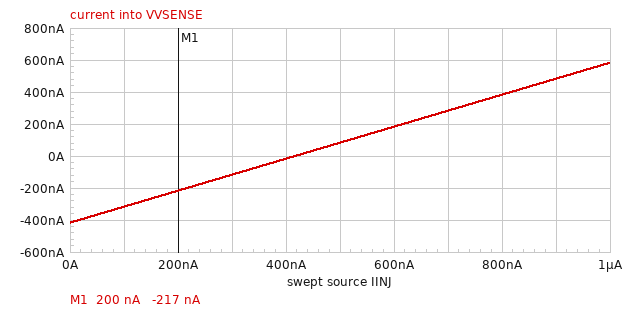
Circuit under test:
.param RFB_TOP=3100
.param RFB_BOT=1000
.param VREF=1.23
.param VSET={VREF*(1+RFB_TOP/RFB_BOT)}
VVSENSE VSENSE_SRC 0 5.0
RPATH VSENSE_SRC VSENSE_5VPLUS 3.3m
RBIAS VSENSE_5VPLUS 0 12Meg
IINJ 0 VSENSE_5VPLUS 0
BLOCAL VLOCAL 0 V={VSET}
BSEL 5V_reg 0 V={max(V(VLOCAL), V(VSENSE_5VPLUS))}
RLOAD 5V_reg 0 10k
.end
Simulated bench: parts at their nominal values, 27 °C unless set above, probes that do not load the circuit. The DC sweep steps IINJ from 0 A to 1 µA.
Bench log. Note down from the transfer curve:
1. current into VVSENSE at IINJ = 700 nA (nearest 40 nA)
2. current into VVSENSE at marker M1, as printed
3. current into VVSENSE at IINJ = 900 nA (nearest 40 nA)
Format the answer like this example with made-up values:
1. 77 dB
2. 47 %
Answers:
1. 280 nA
2. -217 nA
3. 480 nA
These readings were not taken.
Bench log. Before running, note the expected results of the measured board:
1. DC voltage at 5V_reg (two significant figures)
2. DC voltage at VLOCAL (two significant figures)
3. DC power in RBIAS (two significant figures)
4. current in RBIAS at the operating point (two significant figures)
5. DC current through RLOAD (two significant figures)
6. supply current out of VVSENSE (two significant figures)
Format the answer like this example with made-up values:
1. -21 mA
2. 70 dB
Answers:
1. 5.0 V
2. 5.0 V
3. 2.1 µW
4. 420 nA
5. 500 µA
6. 420 nA
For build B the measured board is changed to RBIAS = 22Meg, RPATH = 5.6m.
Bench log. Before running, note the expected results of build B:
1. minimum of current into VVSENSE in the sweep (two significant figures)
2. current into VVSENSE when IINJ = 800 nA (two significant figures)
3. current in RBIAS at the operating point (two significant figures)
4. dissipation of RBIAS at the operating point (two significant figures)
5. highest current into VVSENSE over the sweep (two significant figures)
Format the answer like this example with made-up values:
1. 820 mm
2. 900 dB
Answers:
1. -230 nA
2. 570 nA
3. 230 nA
4. 1.1 µW
5. 770 nA
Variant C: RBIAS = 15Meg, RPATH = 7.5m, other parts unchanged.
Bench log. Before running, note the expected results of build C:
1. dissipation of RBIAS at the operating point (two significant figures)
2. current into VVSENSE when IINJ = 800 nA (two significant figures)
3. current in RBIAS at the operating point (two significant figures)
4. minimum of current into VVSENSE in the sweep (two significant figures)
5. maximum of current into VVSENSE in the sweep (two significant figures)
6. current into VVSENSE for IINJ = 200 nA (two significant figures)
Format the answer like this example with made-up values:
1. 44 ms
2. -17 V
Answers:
1. 1.7 µW
2. 470 nA
3. 330 nA
4. -330 nA
5. 670 nA
6. -130 nA
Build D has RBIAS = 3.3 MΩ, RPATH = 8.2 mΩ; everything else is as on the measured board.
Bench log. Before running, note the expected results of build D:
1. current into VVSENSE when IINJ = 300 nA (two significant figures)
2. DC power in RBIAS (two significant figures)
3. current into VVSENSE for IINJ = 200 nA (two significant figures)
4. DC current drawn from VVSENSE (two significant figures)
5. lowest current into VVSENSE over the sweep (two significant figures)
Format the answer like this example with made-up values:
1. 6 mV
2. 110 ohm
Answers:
1. -1.2 µA
2. 7.6 µW
3. -1.3 µA
4. 1.5 µA
5. -1.5 µA
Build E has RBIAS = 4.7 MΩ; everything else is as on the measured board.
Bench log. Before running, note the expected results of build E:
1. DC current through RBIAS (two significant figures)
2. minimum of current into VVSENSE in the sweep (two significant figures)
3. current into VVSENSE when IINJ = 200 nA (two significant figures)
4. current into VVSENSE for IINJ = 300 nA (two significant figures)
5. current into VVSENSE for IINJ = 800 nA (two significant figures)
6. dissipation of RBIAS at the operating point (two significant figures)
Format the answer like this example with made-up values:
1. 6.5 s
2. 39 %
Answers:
1. 1.1 µA
2. -1.1 µA
3. -860 nA
4. -760 nA
5. -260 nA
6. 5.3 µW
